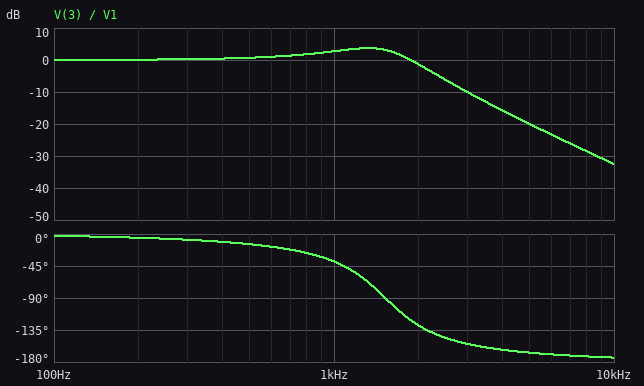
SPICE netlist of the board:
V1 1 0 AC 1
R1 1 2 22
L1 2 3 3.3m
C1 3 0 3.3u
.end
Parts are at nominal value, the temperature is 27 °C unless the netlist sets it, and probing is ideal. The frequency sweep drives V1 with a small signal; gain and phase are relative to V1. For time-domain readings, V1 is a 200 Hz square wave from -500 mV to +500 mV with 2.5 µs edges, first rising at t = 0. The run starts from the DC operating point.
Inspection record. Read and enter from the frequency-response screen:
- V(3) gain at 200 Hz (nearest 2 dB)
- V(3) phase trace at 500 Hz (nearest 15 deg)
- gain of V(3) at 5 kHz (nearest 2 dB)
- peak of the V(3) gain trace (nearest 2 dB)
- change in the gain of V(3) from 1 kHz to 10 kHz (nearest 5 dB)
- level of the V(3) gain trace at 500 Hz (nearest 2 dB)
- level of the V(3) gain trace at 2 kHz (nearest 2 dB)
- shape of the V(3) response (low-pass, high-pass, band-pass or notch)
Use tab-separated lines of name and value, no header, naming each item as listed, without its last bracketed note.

V(3) gain at 200 Hz	0 dB
V(3) phase trace at 500 Hz	-15 deg
gain of V(3) at 5 kHz	-20 dB
peak of the V(3) gain trace	4 dB
change in the gain of V(3) from 1 kHz to 10 kHz	-35 dB
level of the V(3) gain trace at 500 Hz	0 dB
level of the V(3) gain trace at 2 kHz	-2 dB
shape of the V(3) response	low-pass
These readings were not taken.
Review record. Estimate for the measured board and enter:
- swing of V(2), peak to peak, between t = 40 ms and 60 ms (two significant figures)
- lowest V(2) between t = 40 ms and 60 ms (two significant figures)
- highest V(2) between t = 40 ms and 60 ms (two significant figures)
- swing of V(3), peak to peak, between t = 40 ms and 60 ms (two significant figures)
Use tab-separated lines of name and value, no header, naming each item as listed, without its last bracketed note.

swing of V(2), peak to peak, between t = 40 ms and 60 ms	1.3 V
lowest V(2) between t = 40 ms and 60 ms	-640 mV
highest V(2) between t = 40 ms and 60 ms	640 mV
swing of V(3), peak to peak, between t = 40 ms and 60 ms	1.6 V
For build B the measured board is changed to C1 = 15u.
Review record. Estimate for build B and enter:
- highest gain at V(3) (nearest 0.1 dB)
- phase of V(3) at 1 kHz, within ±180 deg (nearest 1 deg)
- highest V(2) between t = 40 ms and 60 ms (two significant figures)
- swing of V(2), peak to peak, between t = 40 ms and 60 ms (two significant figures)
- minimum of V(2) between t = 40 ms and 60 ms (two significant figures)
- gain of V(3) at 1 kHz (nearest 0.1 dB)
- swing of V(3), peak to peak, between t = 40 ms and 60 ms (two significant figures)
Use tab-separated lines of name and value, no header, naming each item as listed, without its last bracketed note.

highest gain at V(3)	0 dB
phase of V(3) at 1 kHz, within ±180 deg	-115 deg
highest V(2) between t = 40 ms and 60 ms	520 mV
swing of V(2), peak to peak, between t = 40 ms and 60 ms	1.0 V
minimum of V(2) between t = 40 ms and 60 ms	-520 mV
gain of V(3) at 1 kHz	-7.2 dB
swing of V(3), peak to peak, between t = 40 ms and 60 ms	1.1 V
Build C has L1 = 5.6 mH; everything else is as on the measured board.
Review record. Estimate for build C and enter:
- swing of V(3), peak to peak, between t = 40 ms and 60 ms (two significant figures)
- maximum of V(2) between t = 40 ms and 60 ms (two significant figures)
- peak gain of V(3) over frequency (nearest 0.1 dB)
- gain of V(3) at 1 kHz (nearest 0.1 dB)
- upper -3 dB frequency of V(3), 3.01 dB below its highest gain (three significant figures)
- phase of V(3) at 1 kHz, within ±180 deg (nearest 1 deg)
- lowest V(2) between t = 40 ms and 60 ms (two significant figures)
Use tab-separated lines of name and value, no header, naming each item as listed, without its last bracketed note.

swing of V(3), peak to peak, between t = 40 ms and 60 ms	1.8 V
maximum of V(2) between t = 40 ms and 60 ms	660 mV
peak gain of V(3) over frequency	5.8 dB
gain of V(3) at 1 kHz	5.5 dB
upper -3 dB frequency of V(3), 3.01 dB below its highest gain	1.37 kHz
phase of V(3) at 1 kHz, within ±180 deg	-59 deg
lowest V(2) between t = 40 ms and 60 ms	-660 mV
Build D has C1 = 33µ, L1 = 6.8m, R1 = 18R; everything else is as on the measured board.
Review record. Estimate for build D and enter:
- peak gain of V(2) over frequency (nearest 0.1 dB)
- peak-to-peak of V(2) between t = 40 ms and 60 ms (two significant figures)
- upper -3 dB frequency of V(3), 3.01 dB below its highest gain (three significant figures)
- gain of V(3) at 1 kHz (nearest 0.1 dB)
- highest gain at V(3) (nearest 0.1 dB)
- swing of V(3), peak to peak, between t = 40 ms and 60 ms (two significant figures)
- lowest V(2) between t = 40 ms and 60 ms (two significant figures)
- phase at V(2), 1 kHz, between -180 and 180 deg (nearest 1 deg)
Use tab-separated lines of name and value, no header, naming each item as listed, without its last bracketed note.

peak gain of V(2) over frequency	0 dB
peak-to-peak of V(2) between t = 40 ms and 60 ms	1.1 V
upper -3 dB frequency of V(3), 3.01 dB below its highest gain	367 Hz
gain of V(3) at 1 kHz	-18.8 dB
highest gain at V(3)	0.2 dB
swing of V(3), peak to peak, between t = 40 ms and 60 ms	1.2 V
lowest V(2) between t = 40 ms and 60 ms	-550 mV
phase at V(2), 1 kHz, between -180 and 180 deg	25 deg
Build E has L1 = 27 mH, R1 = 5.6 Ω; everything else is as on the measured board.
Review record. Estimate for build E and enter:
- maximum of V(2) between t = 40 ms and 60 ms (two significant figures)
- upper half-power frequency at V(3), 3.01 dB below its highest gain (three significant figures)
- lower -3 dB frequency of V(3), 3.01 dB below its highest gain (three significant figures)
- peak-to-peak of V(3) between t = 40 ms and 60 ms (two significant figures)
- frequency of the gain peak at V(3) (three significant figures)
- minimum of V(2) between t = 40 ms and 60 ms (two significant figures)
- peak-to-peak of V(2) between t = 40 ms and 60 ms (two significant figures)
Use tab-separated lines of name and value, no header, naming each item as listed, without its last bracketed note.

maximum of V(2) between t = 40 ms and 60 ms	560 mV
upper half-power frequency at V(3), 3.01 dB below its highest gain	549 Hz
lower -3 dB frequency of V(3), 3.01 dB below its highest gain	516 Hz
peak-to-peak of V(3) between t = 40 ms and 60 ms	2.9 V
frequency of the gain peak at V(3)	533 Hz
minimum of V(2) between t = 40 ms and 60 ms	-560 mV
peak-to-peak of V(2) between t = 40 ms and 60 ms	1.1 V
